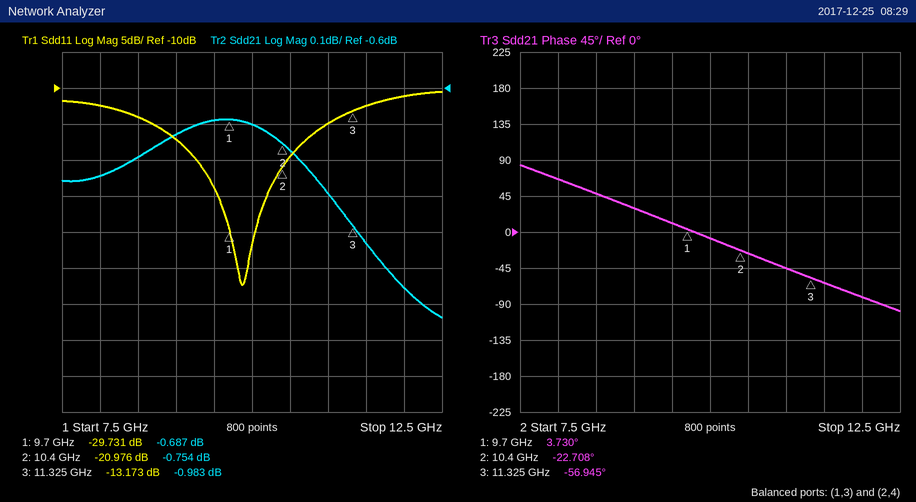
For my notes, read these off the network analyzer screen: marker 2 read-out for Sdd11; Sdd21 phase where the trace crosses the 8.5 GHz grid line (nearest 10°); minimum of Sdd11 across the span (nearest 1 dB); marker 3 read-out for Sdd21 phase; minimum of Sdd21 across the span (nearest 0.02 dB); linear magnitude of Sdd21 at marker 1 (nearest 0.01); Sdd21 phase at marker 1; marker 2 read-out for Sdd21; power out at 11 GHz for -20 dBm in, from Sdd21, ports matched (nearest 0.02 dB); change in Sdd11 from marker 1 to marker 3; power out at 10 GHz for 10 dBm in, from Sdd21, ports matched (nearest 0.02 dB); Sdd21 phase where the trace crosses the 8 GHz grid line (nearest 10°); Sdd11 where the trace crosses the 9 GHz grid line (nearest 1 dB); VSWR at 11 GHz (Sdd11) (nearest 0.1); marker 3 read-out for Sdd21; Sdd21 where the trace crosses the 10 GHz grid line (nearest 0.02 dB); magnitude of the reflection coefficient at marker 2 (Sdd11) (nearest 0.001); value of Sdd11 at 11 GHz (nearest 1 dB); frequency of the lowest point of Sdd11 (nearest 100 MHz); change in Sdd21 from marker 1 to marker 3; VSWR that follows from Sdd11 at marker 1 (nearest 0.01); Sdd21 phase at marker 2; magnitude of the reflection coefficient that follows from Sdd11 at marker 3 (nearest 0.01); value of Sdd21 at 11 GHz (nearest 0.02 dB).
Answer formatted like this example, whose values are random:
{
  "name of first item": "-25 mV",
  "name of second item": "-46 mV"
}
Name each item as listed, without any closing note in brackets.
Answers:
{
  "marker 2 read-out for Sdd11": "-20.976 dB",
  "Sdd21 phase where the trace crosses the 8.5 GHz grid line": "50°",
  "minimum of Sdd11 across the span": "-37 dB",
  "marker 3 read-out for Sdd21 phase": "-56.945°",
  "minimum of Sdd21 across the span": "-1.24 dB",
  "linear magnitude of Sdd21 at marker 1": "0.92",
  "Sdd21 phase at marker 1": "3.730°",
  "marker 2 read-out for Sdd21": "-0.754 dB",
  "power out at 11 GHz for -20 dBm in, from Sdd21, ports matched": "-20.90 dBm",
  "change in Sdd11 from marker 1 to marker 3": "16.558 dB",
  "power out at 10 GHz for 10 dBm in, from Sdd21, ports matched": "9.30 dBm",
  "Sdd21 phase where the trace crosses the 8 GHz grid line": "70°",
  "Sdd11 where the trace crosses the 9 GHz grid line": "-17 dB",
  "VSWR at 11 GHz (Sdd11)": "1.4",
  "marker 3 read-out for Sdd21": "-0.983 dB",
  "Sdd21 where the trace crosses the 10 GHz grid line": "-0.70 dB",
  "magnitude of the reflection coefficient at marker 2 (Sdd11)": "0.089",
  "value of Sdd11 at 11 GHz": "-15 dB",
  "frequency of the lowest point of Sdd11": "9.9 GHz",
  "change in Sdd21 from marker 1 to marker 3": "-0.296 dB",
  "VSWR that follows from Sdd11 at marker 1": "1.07",
  "Sdd21 phase at marker 2": "-22.708°",
  "magnitude of the reflection coefficient that follows from Sdd11 at marker 3": "0.22",
  "value of Sdd21 at 11 GHz": "-0.90 dB"
}
